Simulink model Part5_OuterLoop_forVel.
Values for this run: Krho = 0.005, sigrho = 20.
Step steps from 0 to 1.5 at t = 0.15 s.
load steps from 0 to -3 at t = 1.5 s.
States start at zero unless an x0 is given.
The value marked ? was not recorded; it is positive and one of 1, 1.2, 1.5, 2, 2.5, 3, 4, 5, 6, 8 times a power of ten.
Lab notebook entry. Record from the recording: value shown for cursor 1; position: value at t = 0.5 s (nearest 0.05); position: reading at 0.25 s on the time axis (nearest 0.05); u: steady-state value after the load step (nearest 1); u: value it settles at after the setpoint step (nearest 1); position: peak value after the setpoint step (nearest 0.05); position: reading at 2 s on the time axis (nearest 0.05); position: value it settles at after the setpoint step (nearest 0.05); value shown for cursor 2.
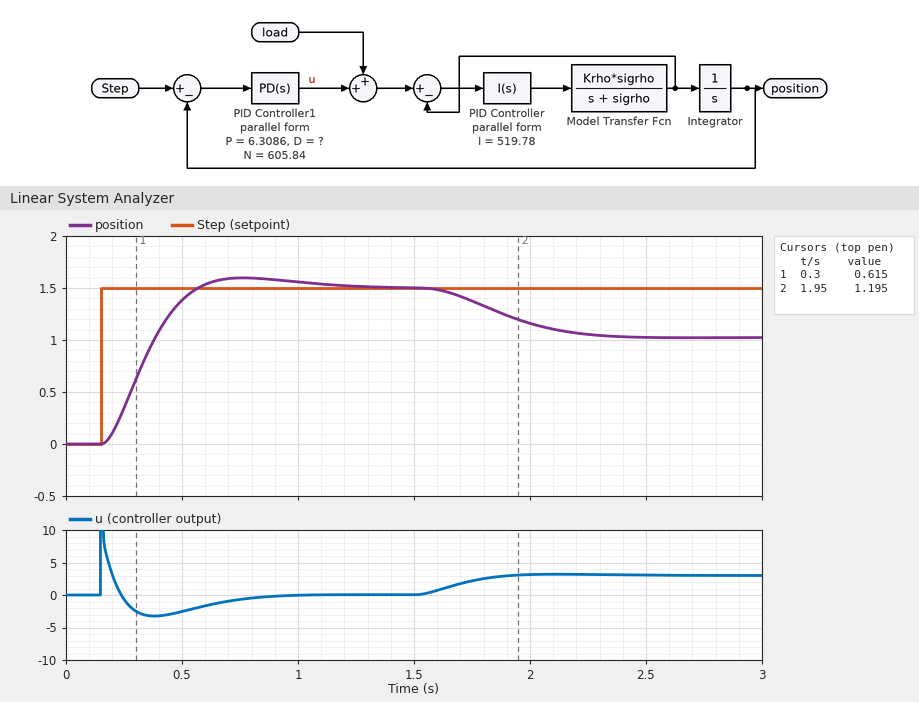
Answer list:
0.615
1.40
0.35
3
0
1.60
1.15
1.50
1.195
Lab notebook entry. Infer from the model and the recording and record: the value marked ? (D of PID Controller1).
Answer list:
1.5
